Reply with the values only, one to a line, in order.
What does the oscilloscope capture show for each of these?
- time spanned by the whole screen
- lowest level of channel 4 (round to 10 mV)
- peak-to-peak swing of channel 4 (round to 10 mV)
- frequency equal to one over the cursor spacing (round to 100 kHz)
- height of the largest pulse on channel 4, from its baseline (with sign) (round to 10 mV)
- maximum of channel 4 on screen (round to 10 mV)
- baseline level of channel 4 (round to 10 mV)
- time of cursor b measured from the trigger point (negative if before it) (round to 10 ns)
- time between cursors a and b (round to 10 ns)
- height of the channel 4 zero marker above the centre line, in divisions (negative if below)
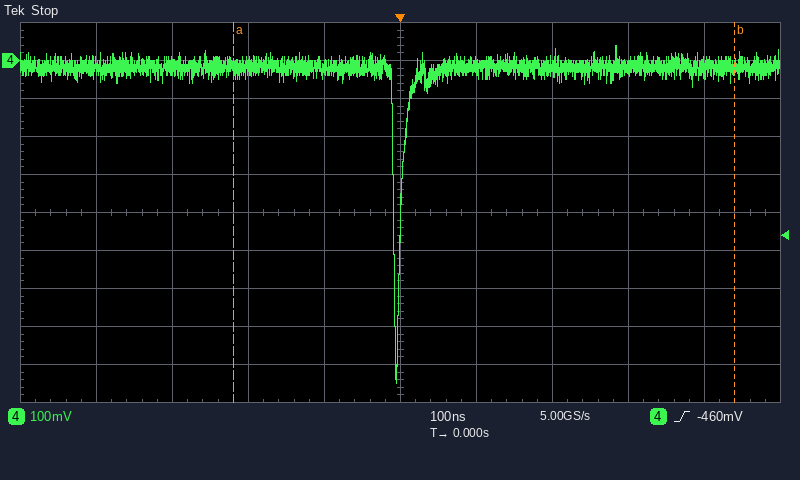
1 µs
-850 mV
890 mV
1.5 MHz
-830 mV
40 mV
-20 mV
+440 ns
660 ns
+4.0 div
